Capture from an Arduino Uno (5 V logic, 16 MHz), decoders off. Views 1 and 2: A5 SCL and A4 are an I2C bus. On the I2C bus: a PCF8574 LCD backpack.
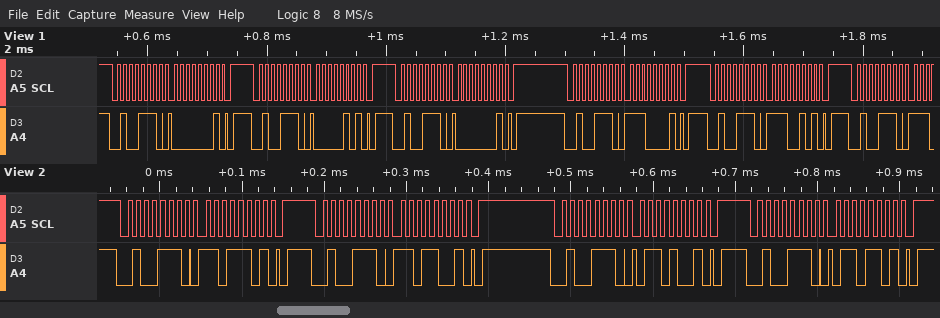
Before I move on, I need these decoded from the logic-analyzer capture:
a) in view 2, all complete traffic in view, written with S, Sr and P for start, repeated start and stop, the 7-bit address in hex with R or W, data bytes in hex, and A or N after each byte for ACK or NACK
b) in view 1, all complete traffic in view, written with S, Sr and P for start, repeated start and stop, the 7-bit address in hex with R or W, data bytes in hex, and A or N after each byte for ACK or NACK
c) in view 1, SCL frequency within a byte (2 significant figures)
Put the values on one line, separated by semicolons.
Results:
S 27W A DD A P S 27W A D9 A P S 27W A 69 A P S 27W A 6D A P; S 27W A 01 A P S 27W A 05 A P S 27W A 01 A P S 27W A E1 A P S 27W A E5 A P S 27W A; 100 kHz
